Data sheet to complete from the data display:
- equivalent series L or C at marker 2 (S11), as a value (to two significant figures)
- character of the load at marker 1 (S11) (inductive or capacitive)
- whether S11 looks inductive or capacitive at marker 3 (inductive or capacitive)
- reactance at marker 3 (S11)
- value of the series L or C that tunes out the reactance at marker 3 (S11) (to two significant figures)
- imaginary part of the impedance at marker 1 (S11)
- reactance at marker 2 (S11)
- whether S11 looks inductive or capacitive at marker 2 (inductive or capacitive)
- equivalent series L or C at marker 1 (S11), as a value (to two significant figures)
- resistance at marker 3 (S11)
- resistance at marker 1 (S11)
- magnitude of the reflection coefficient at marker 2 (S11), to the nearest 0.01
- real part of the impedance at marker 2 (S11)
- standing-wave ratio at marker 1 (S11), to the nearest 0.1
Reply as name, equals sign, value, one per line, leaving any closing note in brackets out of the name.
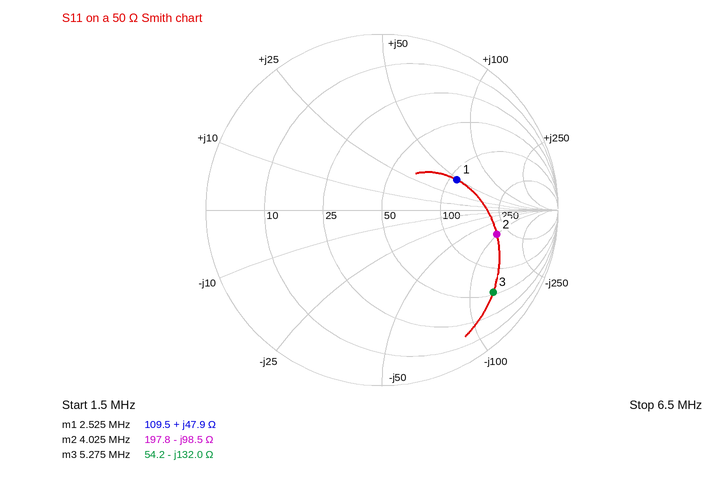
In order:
equivalent series L or C at marker 2 (S11), as a value = 400 pF
character of the load at marker 1 (S11) = inductive
whether S11 looks inductive or capacitive at marker 3 = capacitive
reactance at marker 3 = -132.0 Ω
value of the series L or C that tunes out the reactance at marker 3 (S11) = 4.0 µH
imaginary part of the impedance at marker 1 = +47.9 Ω
reactance at marker 2 = -98.5 Ω
whether S11 looks inductive or capacitive at marker 2 = capacitive
equivalent series L or C at marker 1 (S11), as a value = 3.0 µH
resistance at marker 3 = 54.2 Ω
resistance at marker 1 = 109.5 Ω
magnitude of the reflection coefficient at marker 2 (S11), to the nearest 0.01 = 0.67
real part of the impedance at marker 2 = 197.8 Ω
standing-wave ratio at marker 1 (S11), to the nearest 0.1 = 2.7
